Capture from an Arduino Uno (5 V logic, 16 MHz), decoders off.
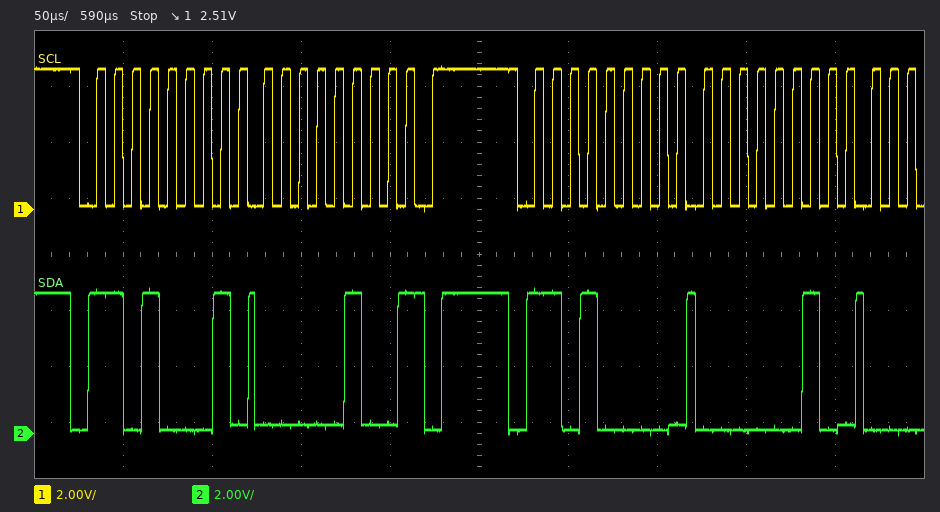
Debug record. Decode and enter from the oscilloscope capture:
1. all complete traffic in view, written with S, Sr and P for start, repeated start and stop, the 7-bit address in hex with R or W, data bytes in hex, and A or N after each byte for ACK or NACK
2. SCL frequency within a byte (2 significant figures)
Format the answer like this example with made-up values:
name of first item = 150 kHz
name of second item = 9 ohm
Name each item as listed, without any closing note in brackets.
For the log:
all complete traffic in view, written with S, Sr and P for start, repeated start and stop, the 7-bit address in hex with R or W, data bytes in hex, and A or N after each byte for ACK or NACK = S 68R A 04 N P S 68W A 02 A
SCL frequency within a byte = 100 kHz
